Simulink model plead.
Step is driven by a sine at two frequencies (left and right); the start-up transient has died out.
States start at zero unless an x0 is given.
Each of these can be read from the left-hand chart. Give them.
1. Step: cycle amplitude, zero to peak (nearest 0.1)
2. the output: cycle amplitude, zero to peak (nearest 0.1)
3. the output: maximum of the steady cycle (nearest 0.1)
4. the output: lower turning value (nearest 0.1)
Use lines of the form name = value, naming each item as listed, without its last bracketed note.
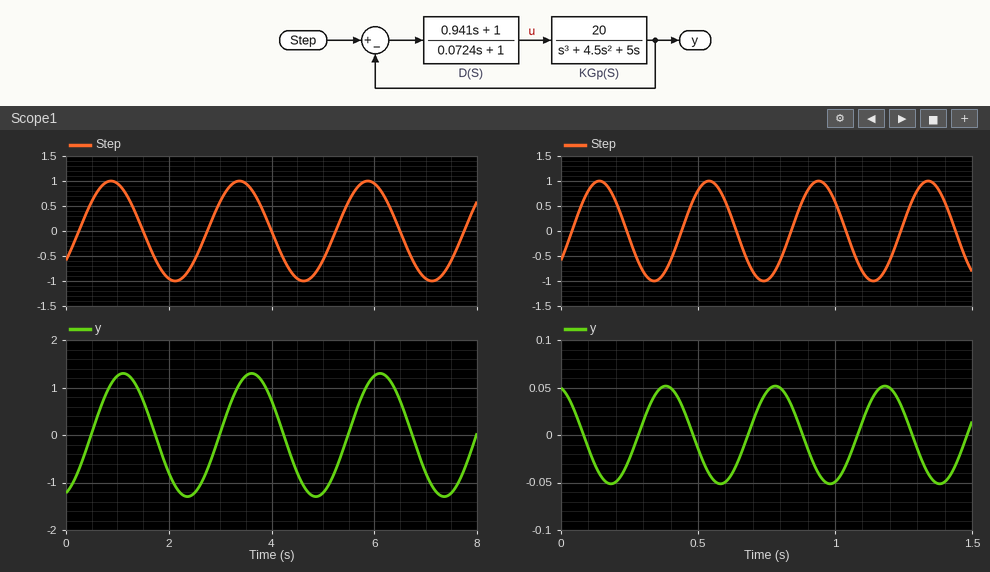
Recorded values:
Step: cycle amplitude, zero to peak = 1.0
the output: cycle amplitude, zero to peak = 1.3
the output: maximum of the steady cycle = 1.3
the output: lower turning value = -1.3
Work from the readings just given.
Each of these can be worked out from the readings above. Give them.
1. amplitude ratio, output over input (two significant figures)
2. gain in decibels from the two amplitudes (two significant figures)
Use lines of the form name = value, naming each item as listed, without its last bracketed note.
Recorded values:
amplitude ratio, output over input = 1.3
gain in decibels from the two amplitudes = 2.3 dB
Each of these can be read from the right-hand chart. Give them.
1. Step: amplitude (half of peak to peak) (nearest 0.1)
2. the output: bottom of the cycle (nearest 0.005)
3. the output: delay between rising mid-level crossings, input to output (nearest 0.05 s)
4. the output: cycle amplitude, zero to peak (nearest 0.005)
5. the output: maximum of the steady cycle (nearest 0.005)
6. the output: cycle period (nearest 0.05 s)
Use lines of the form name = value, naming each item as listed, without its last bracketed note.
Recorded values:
Step: amplitude (half of peak to peak) = 1.0
the output: bottom of the cycle = -0.050
the output: delay between rising mid-level crossings, input to output = 0.25 s
the output: cycle amplitude, zero to peak = 0.050
the output: maximum of the steady cycle = 0.050
the output: cycle period = 0.40 s
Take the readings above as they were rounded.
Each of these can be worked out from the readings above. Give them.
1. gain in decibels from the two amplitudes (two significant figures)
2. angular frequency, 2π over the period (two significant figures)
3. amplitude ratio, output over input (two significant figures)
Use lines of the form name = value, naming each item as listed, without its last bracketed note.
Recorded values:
gain in decibels from the two amplitudes = -26 dB
angular frequency, 2π over the period = 16 rad/s
amplitude ratio, output over input = 0.050
